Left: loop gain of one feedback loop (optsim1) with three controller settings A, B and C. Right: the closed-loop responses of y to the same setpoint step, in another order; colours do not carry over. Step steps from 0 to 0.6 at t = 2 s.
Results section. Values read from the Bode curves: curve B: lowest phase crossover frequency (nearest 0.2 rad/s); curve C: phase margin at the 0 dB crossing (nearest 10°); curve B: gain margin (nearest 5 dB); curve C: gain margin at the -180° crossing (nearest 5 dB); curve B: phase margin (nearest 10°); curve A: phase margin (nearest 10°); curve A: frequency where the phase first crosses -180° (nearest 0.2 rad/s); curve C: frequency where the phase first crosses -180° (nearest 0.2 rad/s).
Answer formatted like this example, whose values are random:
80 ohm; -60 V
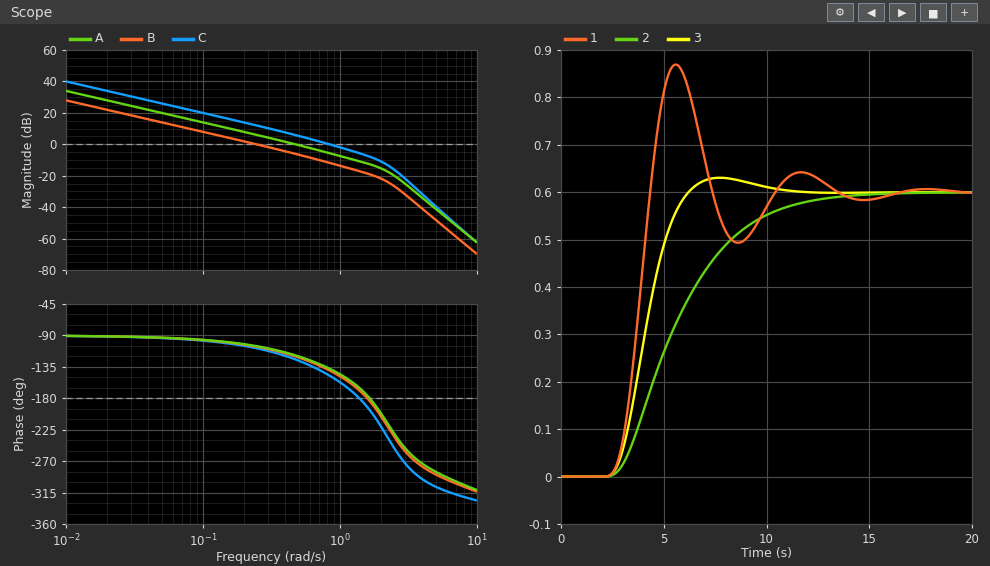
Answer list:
1.6 rad/s; 30°; 20 dB; 5 dB; 70°; 60°; 1.6 rad/s; 1.4 rad/s
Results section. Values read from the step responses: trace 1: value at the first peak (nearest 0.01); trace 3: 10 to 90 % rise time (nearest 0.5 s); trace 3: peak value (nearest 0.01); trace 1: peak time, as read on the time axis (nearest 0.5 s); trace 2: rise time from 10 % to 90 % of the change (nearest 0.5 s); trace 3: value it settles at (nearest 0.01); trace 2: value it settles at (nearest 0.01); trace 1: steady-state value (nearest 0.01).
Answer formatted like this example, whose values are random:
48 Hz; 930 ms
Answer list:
0.87; 2.5 s; 0.63; 5.5 s; 6.0 s; 0.60; 0.60; 0.60
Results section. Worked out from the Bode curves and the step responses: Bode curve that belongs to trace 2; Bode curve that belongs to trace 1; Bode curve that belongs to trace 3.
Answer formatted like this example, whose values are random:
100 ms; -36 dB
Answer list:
B; C; A
